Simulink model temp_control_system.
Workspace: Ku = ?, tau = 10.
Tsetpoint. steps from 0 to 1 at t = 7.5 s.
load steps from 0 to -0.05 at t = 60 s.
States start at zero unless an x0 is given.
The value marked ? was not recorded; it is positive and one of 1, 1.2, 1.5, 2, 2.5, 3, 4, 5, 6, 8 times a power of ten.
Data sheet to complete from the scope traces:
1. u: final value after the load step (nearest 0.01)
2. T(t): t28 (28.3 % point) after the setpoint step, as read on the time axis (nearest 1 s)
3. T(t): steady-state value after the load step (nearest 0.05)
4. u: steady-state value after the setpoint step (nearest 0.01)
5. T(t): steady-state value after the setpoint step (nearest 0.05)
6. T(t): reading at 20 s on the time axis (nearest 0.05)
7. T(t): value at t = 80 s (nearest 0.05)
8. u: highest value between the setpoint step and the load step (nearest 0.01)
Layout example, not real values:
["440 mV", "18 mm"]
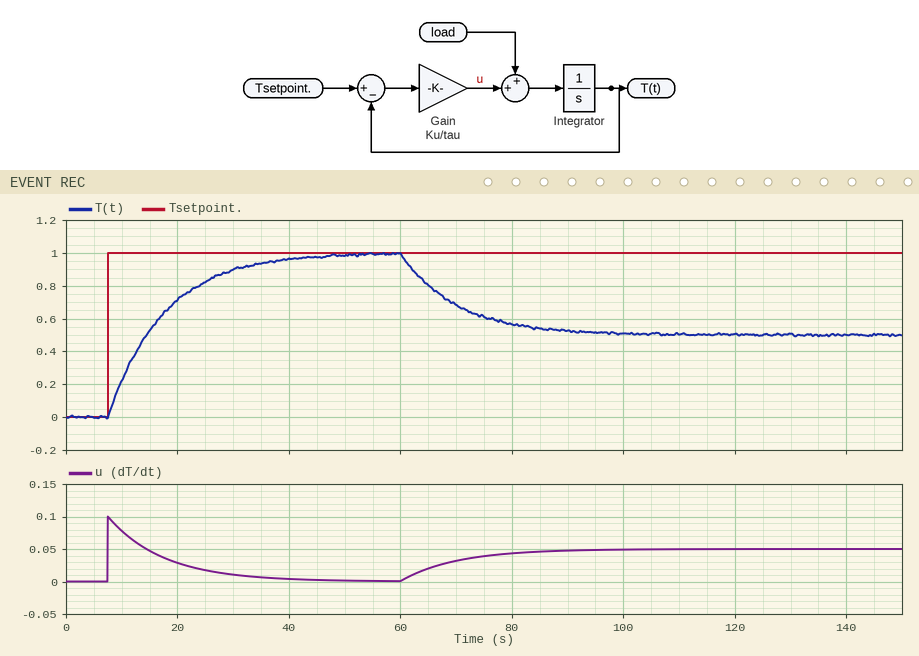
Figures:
["0.05", "11 s", "0.50", "0.00", "1.00", "0.70", "0.55", "0.10"]
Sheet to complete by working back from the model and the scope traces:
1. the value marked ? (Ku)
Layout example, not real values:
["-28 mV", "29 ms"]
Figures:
["1"]
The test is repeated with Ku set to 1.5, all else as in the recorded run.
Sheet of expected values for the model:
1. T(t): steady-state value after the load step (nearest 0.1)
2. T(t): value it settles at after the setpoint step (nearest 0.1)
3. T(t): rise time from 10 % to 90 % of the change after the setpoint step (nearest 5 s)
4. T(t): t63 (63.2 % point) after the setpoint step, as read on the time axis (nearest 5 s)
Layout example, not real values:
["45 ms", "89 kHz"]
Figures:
["0.7", "1.0", "15 s", "15 s"]
